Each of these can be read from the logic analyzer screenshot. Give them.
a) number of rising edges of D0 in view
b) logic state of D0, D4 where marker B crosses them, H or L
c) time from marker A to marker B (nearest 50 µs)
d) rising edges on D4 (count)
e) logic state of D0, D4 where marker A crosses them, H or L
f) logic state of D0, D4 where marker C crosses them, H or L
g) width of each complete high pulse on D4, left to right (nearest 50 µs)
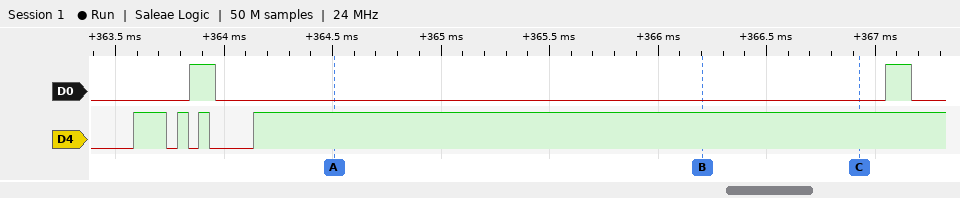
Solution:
2
D0=L, D4=H
1700 µs
4
D0=L, D4=H
D0=L, D4=H
150 µs, 50 µs, 50 µs
